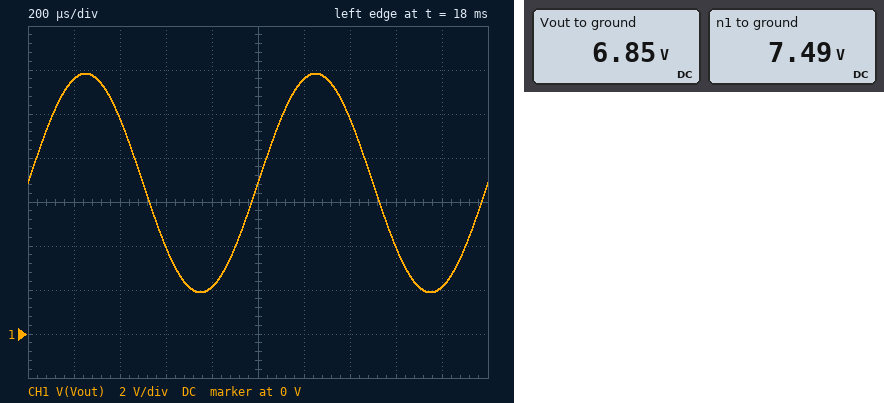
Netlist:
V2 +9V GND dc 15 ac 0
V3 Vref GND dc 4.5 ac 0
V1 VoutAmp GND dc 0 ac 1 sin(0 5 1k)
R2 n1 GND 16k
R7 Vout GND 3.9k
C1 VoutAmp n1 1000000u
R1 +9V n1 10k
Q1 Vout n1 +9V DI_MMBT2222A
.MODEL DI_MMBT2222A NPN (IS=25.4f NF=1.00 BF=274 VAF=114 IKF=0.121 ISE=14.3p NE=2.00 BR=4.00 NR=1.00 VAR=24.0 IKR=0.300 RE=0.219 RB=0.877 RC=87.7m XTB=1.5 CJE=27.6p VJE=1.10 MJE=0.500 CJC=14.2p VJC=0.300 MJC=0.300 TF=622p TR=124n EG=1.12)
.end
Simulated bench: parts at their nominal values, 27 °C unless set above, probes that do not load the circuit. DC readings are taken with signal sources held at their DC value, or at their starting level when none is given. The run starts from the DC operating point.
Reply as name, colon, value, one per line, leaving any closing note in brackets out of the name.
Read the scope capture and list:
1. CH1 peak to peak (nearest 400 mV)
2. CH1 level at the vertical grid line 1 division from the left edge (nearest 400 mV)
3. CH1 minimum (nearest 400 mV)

CH1 peak to peak: 10.0 V
CH1 level at the vertical grid line 1 division from the left edge: 11.6 V
CH1 minimum: 2.0 V
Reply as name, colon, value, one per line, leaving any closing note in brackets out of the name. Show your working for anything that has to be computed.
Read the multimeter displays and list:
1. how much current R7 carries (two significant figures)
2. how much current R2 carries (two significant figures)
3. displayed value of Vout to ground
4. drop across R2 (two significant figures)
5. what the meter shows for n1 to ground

how much current R7 carries: (6.85 V) / 3.9 kΩ = 1.8 mA
how much current R2 carries: (7.49 V) / 16 kΩ = 470 µA
displayed value of Vout to ground: 6.85 V
drop across R2: 7.49 V = 7.5 V
what the meter shows for n1 to ground: 7.49 V
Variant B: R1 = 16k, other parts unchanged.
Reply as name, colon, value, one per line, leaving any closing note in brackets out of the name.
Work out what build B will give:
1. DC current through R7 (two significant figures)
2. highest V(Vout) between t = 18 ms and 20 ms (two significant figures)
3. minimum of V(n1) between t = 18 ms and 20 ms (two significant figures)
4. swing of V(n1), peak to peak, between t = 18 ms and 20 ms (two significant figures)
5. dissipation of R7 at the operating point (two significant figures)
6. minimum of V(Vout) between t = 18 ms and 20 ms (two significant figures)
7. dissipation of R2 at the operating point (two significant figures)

DC current through R7: 1.3 mA
highest V(Vout) between t = 18 ms and 20 ms: 10 V
minimum of V(n1) between t = 18 ms and 20 ms: 850 mV
swing of V(n1), peak to peak, between t = 18 ms and 20 ms: 10 V
dissipation of R7 at the operating point: 7.0 mW
minimum of V(Vout) between t = 18 ms and 20 ms: 300 mV
dissipation of R2 at the operating point: 2.1 mW
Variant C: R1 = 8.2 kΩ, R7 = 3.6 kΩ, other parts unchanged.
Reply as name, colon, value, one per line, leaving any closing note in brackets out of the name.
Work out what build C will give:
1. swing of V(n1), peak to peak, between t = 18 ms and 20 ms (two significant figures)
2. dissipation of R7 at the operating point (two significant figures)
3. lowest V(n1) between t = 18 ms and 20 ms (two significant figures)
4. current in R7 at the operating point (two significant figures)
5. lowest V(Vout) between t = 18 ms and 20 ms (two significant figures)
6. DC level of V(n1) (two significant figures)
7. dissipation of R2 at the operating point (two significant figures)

swing of V(n1), peak to peak, between t = 18 ms and 20 ms: 10 V
dissipation of R7 at the operating point: 15 mW
lowest V(n1) between t = 18 ms and 20 ms: 3.1 V
current in R7 at the operating point: 2.1 mA
lowest V(Vout) between t = 18 ms and 20 ms: 2.5 V
DC level of V(n1): 8.1 V
dissipation of R2 at the operating point: 4.1 mW
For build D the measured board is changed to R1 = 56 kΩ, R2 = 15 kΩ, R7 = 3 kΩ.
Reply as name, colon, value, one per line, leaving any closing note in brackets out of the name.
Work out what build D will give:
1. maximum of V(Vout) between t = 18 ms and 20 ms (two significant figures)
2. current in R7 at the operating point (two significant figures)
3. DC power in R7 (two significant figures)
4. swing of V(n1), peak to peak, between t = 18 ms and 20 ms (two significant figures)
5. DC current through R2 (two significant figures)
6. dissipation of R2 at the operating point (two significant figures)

maximum of V(Vout) between t = 18 ms and 20 ms: 6.6 V
current in R7 at the operating point: 550 µA
DC power in R7: 910 µW
swing of V(n1), peak to peak, between t = 18 ms and 20 ms: 10 V
DC current through R2: 150 µA
dissipation of R2 at the operating point: 340 µW
